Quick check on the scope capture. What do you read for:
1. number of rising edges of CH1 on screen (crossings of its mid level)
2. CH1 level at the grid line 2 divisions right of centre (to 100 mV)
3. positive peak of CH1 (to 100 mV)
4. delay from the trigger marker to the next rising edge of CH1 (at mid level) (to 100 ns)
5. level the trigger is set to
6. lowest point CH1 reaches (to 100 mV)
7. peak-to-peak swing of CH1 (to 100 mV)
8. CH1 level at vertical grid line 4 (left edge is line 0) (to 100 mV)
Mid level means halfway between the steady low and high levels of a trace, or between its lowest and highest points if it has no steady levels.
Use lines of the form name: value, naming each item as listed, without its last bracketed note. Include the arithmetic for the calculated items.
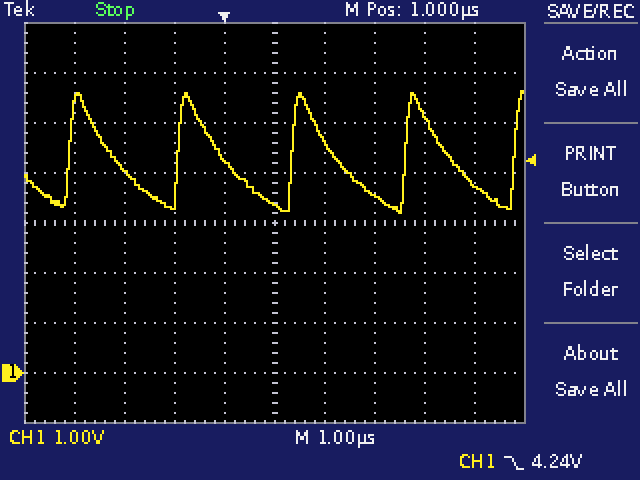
number of rising edges of CH1 on screen: 5
CH1 level at the grid line 2 divisions right of centre: 3.6 V
positive peak of CH1: 5.6 V
delay from the trigger marker to the next rising edge of CH1 (at mid level): 1.4 µs
level the trigger is set to: 4.24 V
lowest point CH1 reaches: 3.2 V
peak-to-peak swing of CH1: 5.6 V − (3.2 V) = 2.4 V
CH1 level at vertical grid line 4 (left edge is line 0): 4.3 V
